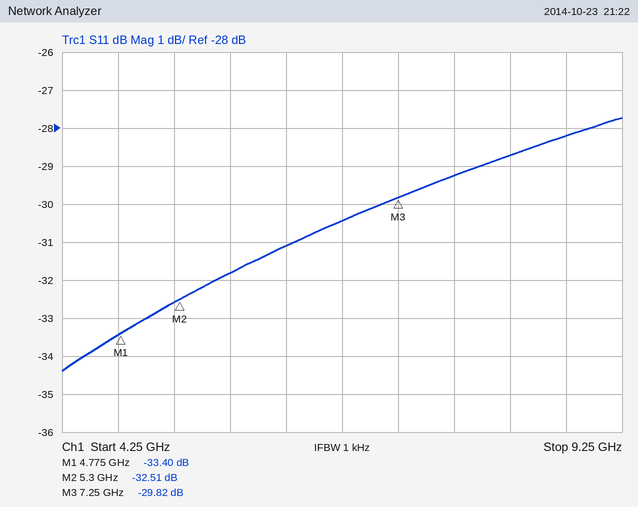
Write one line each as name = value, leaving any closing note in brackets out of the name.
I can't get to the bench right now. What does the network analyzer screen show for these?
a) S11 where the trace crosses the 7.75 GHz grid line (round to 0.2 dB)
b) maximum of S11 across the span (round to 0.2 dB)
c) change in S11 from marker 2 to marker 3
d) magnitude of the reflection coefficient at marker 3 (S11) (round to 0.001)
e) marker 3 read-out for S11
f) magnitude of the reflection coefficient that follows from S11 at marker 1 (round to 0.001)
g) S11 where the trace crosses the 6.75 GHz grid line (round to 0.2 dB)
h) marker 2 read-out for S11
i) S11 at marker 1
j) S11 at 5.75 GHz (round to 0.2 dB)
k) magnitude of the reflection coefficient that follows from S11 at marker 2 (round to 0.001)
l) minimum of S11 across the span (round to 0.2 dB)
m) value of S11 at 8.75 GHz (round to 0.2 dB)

S11 where the trace crosses the 7.75 GHz grid line = -29.2 dB
maximum of S11 across the span = -27.8 dB
change in S11 from marker 2 to marker 3 = 2.69 dB
magnitude of the reflection coefficient at marker 3 (S11) = 0.032
marker 3 read-out for S11 = -29.82 dB
magnitude of the reflection coefficient that follows from S11 at marker 1 = 0.021
S11 where the trace crosses the 6.75 GHz grid line = -30.4 dB
marker 2 read-out for S11 = -32.51 dB
S11 at marker 1 = -33.40 dB
S11 at 5.75 GHz = -31.8 dB
magnitude of the reflection coefficient that follows from S11 at marker 2 = 0.024
minimum of S11 across the span = -34.4 dB
value of S11 at 8.75 GHz = -28.2 dB
